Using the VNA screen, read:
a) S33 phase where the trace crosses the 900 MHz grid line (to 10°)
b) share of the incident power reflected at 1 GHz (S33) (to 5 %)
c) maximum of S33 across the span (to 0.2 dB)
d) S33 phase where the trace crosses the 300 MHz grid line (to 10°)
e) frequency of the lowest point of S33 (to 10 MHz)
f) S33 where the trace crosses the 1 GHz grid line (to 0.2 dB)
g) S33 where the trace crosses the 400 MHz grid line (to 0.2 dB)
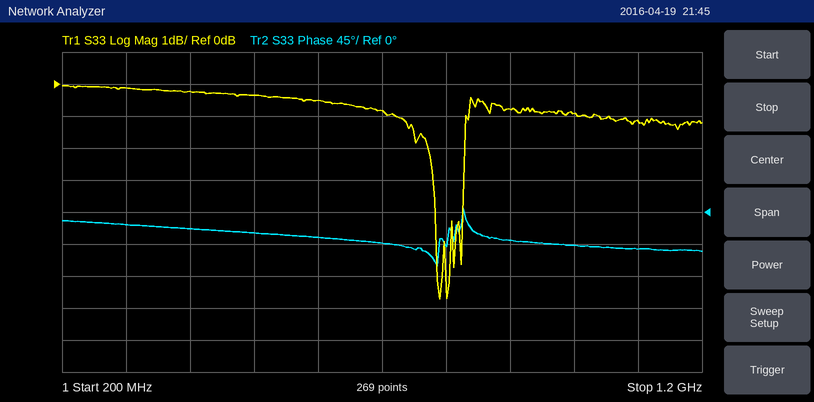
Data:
-40°
80 %
0.0 dB
-20°
790 MHz
-1.0 dB
-0.2 dB
